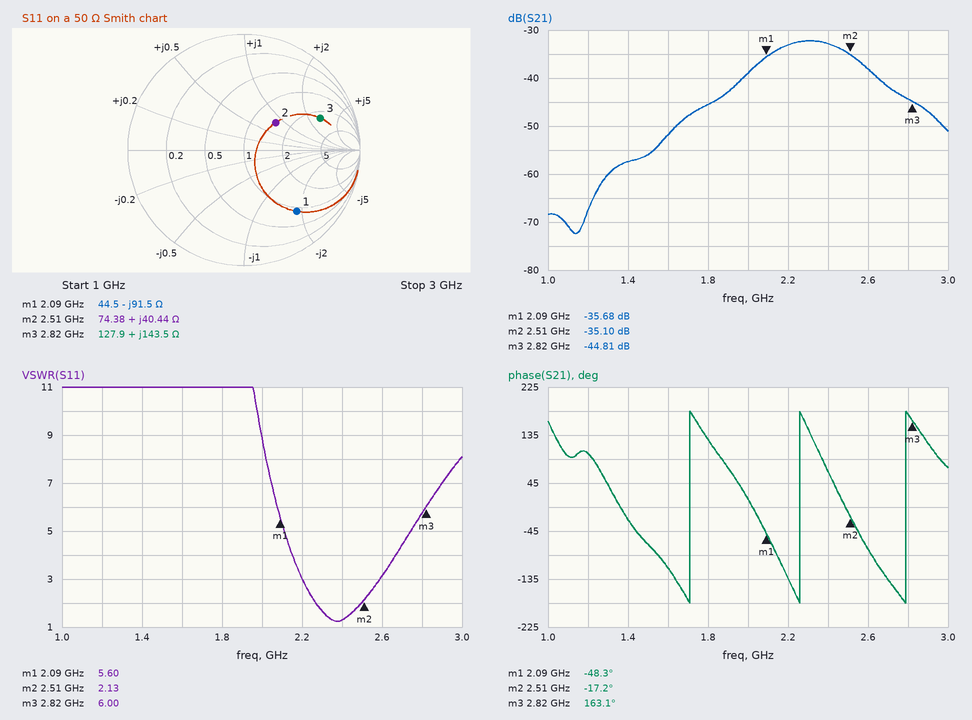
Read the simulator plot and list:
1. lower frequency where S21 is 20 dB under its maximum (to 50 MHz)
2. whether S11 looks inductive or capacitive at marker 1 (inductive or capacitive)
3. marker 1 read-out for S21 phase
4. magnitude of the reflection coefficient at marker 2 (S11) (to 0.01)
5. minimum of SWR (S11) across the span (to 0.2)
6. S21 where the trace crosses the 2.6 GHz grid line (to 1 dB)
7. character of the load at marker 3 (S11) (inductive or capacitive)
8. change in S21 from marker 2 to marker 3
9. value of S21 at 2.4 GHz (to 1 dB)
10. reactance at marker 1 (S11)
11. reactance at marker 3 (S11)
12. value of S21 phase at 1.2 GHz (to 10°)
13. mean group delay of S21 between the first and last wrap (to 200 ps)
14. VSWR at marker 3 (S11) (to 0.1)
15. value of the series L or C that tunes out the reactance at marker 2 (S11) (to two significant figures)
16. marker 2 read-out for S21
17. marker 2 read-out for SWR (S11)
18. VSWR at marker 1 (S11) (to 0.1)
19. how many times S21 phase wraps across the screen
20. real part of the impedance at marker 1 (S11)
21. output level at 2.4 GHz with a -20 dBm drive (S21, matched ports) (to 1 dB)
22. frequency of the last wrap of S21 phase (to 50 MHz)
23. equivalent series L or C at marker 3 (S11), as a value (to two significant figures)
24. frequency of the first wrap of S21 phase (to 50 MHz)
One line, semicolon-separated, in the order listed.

1.60 GHz; capacitive; -48.3°; 0.36; 1.2; -38 dB; inductive; -9.71 dB; -33 dB; -91.5 Ω; +143.5 Ω; 100°; 1.8 ns; 6.0; 1.6 pF; -35.10 dB; 2.13; 5.6; 3; 44.5 Ω; -53 dBm; 2.80 GHz; 8.1 nH; 1.70 GHz
